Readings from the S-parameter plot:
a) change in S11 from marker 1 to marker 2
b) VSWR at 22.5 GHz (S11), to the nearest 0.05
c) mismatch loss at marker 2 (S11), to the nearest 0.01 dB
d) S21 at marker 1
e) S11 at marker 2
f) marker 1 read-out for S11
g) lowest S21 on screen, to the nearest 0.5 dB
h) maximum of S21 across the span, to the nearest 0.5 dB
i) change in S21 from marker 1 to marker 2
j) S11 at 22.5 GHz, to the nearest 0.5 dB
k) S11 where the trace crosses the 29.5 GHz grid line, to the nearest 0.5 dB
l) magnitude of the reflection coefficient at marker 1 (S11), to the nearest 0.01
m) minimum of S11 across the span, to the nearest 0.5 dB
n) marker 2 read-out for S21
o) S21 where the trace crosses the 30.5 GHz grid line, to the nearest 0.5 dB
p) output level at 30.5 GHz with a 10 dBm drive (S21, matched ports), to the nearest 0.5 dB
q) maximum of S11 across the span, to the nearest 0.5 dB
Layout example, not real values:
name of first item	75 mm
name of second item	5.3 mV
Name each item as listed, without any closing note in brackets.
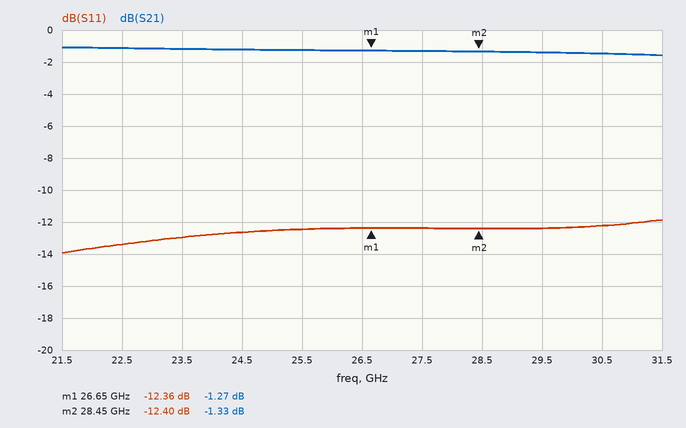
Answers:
change in S11 from marker 1 to marker 2	-0.04 dB
VSWR at 22.5 GHz (S11), to the nearest 0.05	1.55
mismatch loss at marker 2 (S11), to the nearest 0.01 dB	0.26 dB
S21 at marker 1	-1.27 dB
S11 at marker 2	-12.40 dB
marker 1 read-out for S11	-12.36 dB
lowest S21 on screen, to the nearest 0.5 dB	-1.5 dB
maximum of S21 across the span, to the nearest 0.5 dB	-1.0 dB
change in S21 from marker 1 to marker 2	-0.06 dB
S11 at 22.5 GHz, to the nearest 0.5 dB	-13.5 dB
S11 where the trace crosses the 29.5 GHz grid line, to the nearest 0.5 dB	-12.5 dB
magnitude of the reflection coefficient at marker 1 (S11), to the nearest 0.01	0.24
minimum of S11 across the span, to the nearest 0.5 dB	-14.0 dB
marker 2 read-out for S21	-1.33 dB
S21 where the trace crosses the 30.5 GHz grid line, to the nearest 0.5 dB	-1.5 dB
output level at 30.5 GHz with a 10 dBm drive (S21, matched ports), to the nearest 0.5 dB	8.5 dBm
maximum of S11 across the span, to the nearest 0.5 dB	-12.0 dB
